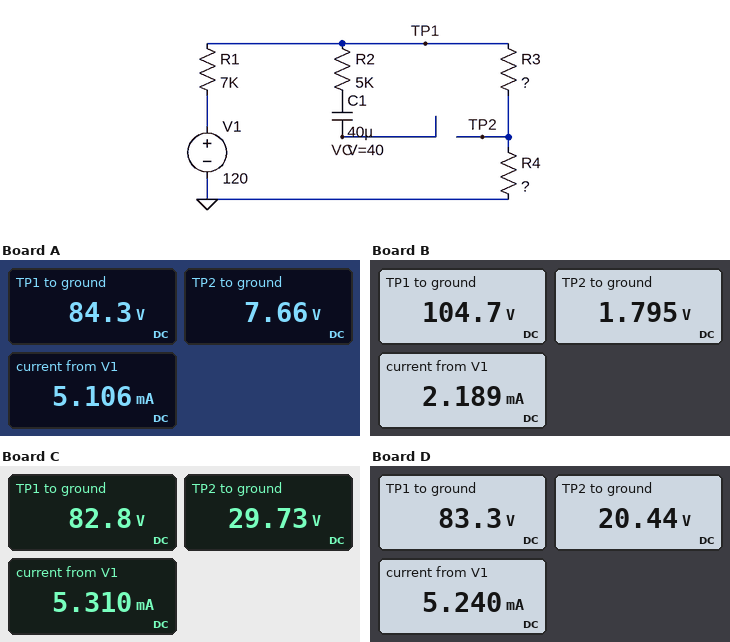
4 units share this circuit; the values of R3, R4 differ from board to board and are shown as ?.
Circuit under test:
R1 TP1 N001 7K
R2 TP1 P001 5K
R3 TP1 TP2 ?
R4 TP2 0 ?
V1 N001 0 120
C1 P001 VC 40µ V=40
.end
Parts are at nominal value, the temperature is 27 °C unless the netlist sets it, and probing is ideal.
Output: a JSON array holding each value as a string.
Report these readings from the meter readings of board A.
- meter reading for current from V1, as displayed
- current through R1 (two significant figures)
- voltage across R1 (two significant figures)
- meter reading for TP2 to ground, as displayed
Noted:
["5.106 mA", "5.1 mA", "36 V", "7.66 V"]
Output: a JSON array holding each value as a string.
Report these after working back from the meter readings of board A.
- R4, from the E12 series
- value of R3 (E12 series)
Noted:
["1.5 kΩ", "15 kΩ"]
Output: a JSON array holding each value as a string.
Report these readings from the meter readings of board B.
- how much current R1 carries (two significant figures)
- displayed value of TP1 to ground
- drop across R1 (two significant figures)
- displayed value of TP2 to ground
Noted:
["2.2 mA", "104.7 V", "15 V", "1.795 V"]
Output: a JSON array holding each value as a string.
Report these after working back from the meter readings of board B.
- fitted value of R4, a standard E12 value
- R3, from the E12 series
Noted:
["820 Ω", "47 kΩ"]
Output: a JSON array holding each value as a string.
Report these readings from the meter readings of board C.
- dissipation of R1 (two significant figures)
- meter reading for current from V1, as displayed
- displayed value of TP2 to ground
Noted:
["200 mW", "5.310 mA", "29.73 V"]
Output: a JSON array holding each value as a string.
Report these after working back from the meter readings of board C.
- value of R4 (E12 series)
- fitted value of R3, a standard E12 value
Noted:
["5.6 kΩ", "10 kΩ"]
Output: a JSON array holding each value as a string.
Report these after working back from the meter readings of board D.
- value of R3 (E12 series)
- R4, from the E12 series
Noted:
["12 kΩ", "3.9 kΩ"]
